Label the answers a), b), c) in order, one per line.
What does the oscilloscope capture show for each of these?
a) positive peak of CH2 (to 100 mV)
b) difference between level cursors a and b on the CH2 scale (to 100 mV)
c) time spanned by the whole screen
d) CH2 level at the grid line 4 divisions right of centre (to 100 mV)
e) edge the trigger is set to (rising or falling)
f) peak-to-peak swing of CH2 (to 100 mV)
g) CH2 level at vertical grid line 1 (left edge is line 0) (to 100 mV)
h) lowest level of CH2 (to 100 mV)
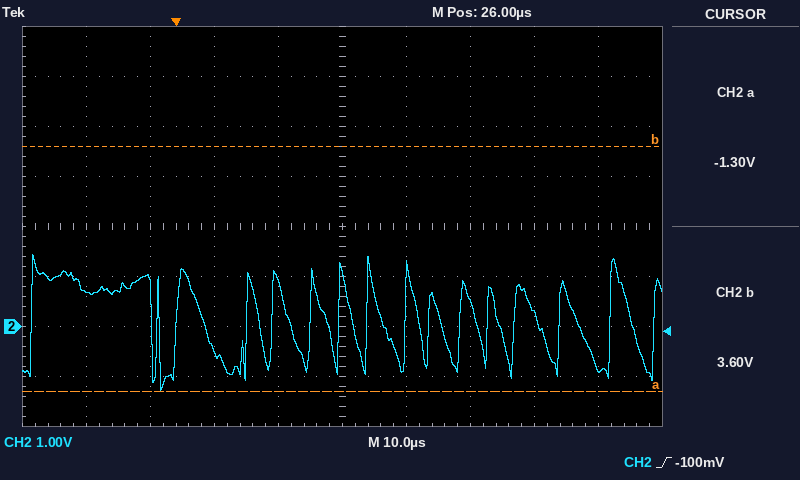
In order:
a) 1.4 V
b) 4.9 V
c) 100 µs
d) -800 mV
e) rising
f) 2.7 V
g) 700 mV
h) -1.3 V
